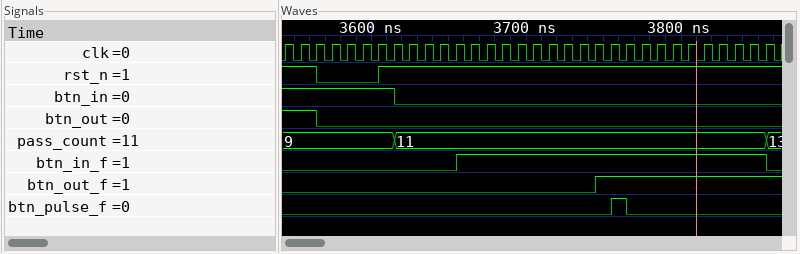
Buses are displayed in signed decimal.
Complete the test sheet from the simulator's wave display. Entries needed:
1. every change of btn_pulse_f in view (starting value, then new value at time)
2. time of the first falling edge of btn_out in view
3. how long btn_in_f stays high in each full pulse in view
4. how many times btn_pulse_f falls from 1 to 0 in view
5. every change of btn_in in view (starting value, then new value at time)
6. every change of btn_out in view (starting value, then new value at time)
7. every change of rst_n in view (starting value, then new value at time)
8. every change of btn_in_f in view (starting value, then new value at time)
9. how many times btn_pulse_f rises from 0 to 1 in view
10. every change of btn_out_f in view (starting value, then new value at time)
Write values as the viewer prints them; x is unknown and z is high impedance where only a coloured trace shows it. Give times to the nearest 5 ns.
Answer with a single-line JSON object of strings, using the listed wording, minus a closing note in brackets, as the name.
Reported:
{"every change of btn_pulse_f in view": "0, 1 at 3755 ns, 0 at 3765 ns", "time of the first falling edge of btn_out in view": "3565 ns", "how long btn_in_f stays high in each full pulse in view": "200 ns", "how many times btn_pulse_f falls from 1 to 0 in view": "1", "every change of btn_in in view": "1, 0 at 3615 ns", "every change of btn_out in view": "1, 0 at 3565 ns", "every change of rst_n in view": "1, 0 at 3565 ns, 1 at 3605 ns", "every change of btn_in_f in view": "0, 1 at 3655 ns, 0 at 3855 ns", "how many times btn_pulse_f rises from 0 to 1 in view": "1", "every change of btn_out_f in view": "0, 1 at 3745 ns"}
